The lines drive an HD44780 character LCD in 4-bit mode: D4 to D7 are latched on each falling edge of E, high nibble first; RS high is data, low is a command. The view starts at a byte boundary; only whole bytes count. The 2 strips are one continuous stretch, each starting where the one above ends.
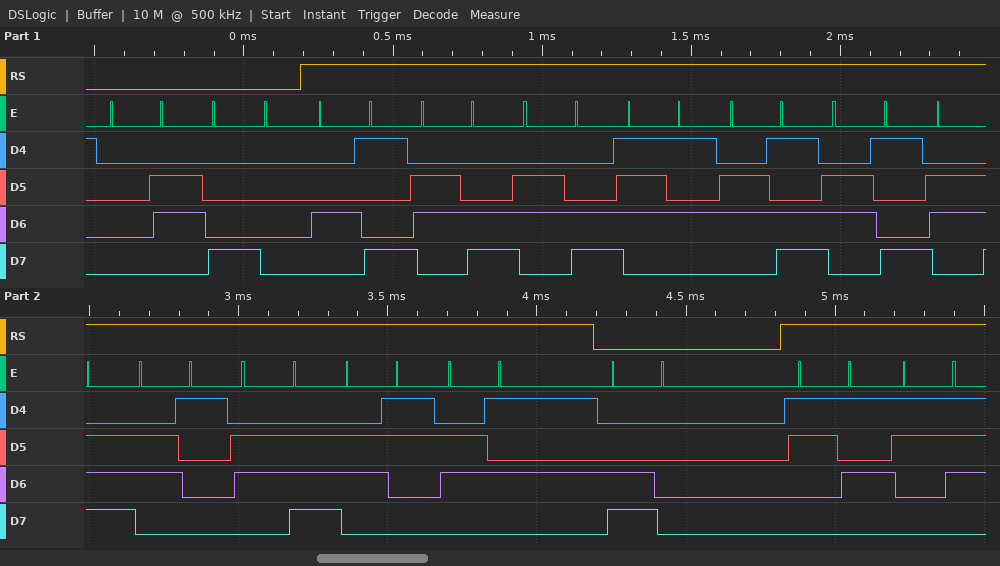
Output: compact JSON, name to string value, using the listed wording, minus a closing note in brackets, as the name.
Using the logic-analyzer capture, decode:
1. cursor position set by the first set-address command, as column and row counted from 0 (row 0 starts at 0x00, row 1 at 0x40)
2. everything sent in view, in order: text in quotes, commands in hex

{"cursor position set by the first set-address command, as column and row counted from 0": "column 0, row 0", "everything sent in view, in order: text in quotes, commands in hex": "0x06 0x80 \"Illuminance\" 0xC0 \"57\""}
